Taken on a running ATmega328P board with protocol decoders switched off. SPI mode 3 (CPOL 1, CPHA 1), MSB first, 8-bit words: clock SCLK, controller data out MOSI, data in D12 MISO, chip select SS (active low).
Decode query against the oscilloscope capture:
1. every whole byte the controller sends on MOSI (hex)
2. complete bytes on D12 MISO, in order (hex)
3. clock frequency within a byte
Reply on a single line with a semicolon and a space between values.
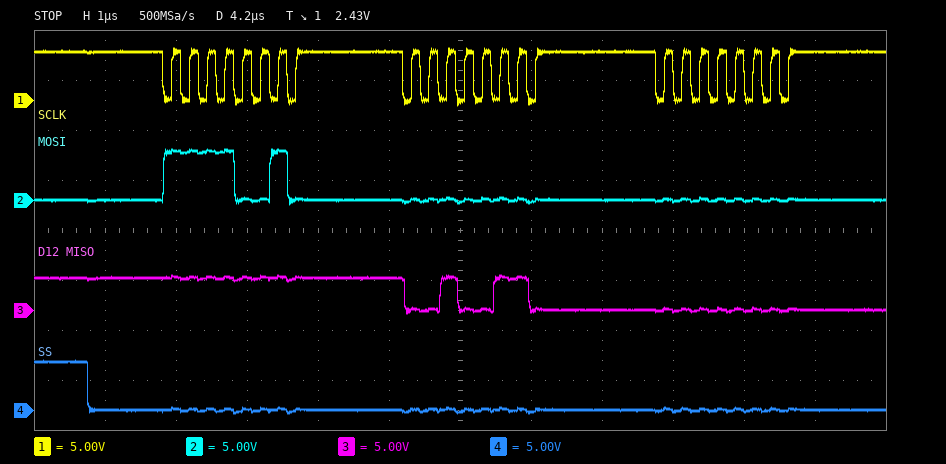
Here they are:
F2 00 00; FF 26 00; 4 MHz
